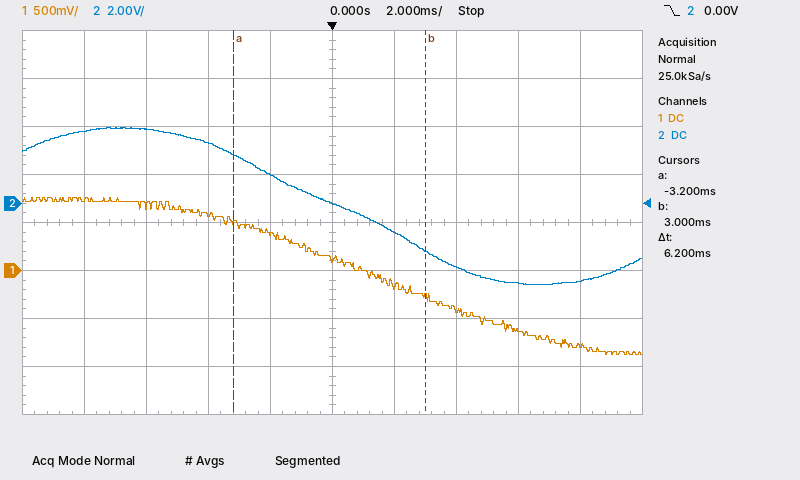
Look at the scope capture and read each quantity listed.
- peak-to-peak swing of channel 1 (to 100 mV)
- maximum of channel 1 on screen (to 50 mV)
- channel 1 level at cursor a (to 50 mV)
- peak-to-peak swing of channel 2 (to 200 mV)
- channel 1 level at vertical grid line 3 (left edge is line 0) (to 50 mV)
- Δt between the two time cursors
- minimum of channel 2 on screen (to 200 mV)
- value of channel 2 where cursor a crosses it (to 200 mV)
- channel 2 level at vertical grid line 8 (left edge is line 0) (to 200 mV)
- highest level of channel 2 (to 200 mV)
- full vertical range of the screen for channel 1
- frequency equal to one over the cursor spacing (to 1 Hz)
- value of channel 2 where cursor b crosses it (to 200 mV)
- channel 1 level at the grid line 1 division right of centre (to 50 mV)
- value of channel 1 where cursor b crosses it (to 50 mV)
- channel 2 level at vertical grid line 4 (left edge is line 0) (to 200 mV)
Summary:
1.60 V
750 mV
500 mV
6.6 V
600 mV
6.2 ms
-3.4 V
2.0 V
-3.4 V
3.2 V
4 V
161 Hz
-2.0 V
-150 mV
-300 mV
1.2 V
